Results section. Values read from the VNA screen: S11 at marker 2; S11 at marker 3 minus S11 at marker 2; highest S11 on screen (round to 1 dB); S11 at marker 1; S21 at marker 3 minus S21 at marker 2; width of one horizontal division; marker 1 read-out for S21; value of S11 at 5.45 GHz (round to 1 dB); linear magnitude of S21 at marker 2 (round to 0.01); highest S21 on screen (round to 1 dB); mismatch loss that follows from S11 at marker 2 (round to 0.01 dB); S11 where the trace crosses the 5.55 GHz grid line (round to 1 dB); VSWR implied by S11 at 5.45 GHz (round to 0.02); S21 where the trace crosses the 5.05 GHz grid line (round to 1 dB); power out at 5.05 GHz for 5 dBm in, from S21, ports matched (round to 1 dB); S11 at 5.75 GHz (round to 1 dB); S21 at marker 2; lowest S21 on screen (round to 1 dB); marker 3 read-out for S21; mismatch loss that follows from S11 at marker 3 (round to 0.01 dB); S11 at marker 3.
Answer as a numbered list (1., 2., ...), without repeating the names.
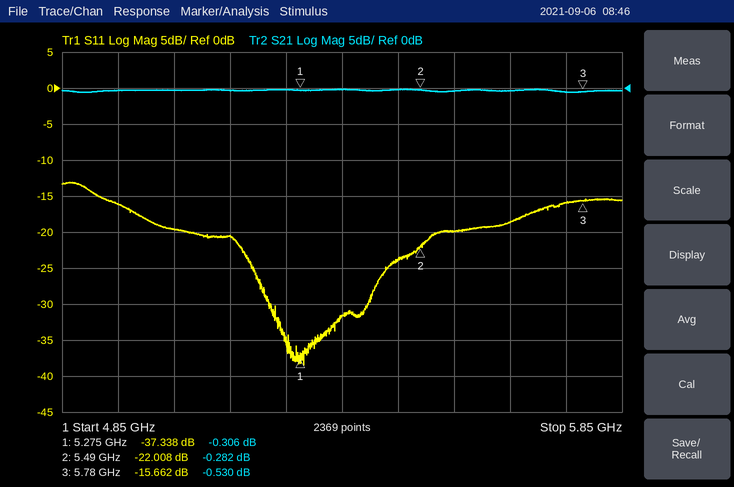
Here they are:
1. -22.008 dB
2. 6.346 dB
3. -13 dB
4. -37.338 dB
5. -0.248 dB
6. 100 MHz
7. -0.306 dB
8. -24 dB
9. 0.97
10. 0 dB
11. 0.03 dB
12. -20 dB
13. 1.14
14. 0 dB
15. 5 dBm
16. -16 dB
17. -0.282 dB
18. -1 dB
19. -0.530 dB
20. 0.12 dB
21. -15.662 dB
